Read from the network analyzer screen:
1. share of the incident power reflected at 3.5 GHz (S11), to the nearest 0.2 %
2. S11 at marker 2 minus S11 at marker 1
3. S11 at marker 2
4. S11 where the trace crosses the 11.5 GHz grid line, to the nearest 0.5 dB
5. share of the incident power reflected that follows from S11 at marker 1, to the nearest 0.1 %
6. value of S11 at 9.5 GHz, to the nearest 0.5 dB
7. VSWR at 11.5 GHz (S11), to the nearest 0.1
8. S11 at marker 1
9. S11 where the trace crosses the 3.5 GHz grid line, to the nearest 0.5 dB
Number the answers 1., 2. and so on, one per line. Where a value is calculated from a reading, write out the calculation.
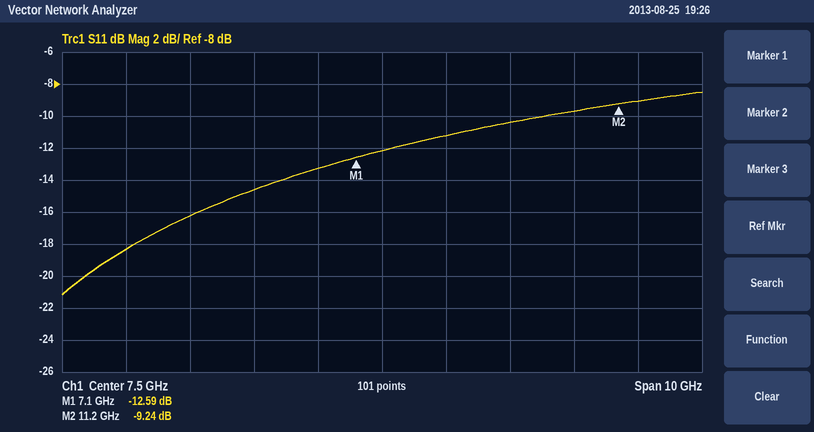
1. 10^(-18.5/10) ≈ 1.4 %
2. -9.24 − (-12.59) = 3.35 dB
3. -9.24 dB
4. -9.0 dB
5. 10^(-12.59/10) ≈ 5.5 %
6. -10.5 dB
7. |Γ| = 10^(-9/20) = 0.3548; VSWR = (1 + 0.3548)/(1 − 0.3548) ≈ 2.1
8. -12.59 dB
9. -18.5 dB
